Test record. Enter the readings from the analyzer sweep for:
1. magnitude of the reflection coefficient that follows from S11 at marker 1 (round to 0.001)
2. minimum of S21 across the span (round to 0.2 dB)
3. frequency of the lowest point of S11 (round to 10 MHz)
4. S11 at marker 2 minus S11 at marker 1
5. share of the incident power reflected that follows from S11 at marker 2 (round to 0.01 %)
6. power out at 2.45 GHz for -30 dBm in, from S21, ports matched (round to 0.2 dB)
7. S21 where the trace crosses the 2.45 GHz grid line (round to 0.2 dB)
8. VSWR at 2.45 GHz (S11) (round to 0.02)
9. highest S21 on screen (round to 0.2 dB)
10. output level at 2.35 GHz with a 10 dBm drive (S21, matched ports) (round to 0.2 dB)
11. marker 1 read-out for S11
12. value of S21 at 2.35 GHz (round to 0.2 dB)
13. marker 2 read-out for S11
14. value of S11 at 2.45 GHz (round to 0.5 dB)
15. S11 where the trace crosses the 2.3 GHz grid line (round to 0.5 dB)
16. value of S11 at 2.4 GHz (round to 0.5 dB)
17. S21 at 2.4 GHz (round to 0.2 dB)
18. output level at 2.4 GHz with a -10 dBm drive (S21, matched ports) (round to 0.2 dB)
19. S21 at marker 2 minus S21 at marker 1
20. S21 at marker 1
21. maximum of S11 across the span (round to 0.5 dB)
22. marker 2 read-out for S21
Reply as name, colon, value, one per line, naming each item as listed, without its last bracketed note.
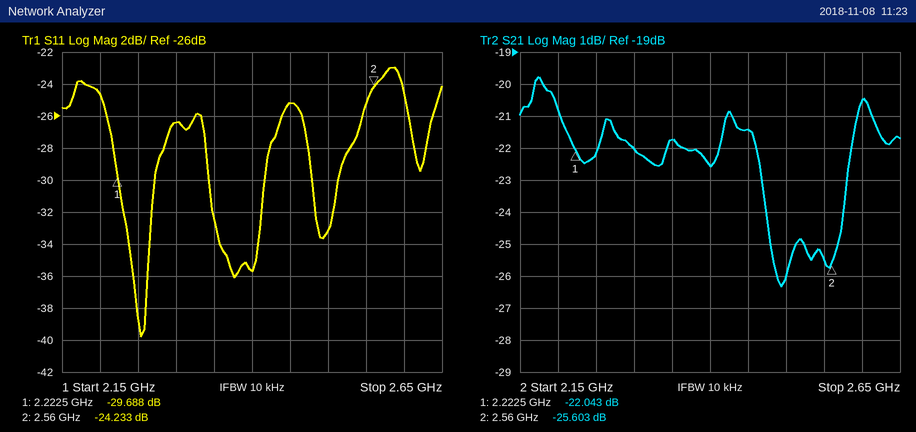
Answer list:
magnitude of the reflection coefficient that follows from S11 at marker 1: 0.033
minimum of S21 across the span: -26.4 dB
frequency of the lowest point of S11: 2.25 GHz
S11 at marker 2 minus S11 at marker 1: 5.455 dB
share of the incident power reflected that follows from S11 at marker 2: 0.38 %
power out at 2.45 GHz for -30 dBm in, from S21, ports matched: -51.4 dBm
S21 where the trace crosses the 2.45 GHz grid line: -21.4 dB
VSWR at 2.45 GHz (S11): 1.12
highest S21 on screen: -19.8 dB
output level at 2.35 GHz with a 10 dBm drive (S21, matched ports): -11.8 dBm
marker 1 read-out for S11: -29.688 dB
value of S21 at 2.35 GHz: -21.8 dB
marker 2 read-out for S11: -24.233 dB
value of S11 at 2.45 GHz: -25.0 dB
S11 where the trace crosses the 2.3 GHz grid line: -26.5 dB
value of S11 at 2.4 GHz: -35.5 dB
S21 at 2.4 GHz: -22.6 dB
output level at 2.4 GHz with a -10 dBm drive (S21, matched ports): -32.6 dBm
S21 at marker 2 minus S21 at marker 1: -3.560 dB
S21 at marker 1: -22.043 dB
maximum of S11 across the span: -23.0 dB
marker 2 read-out for S21: -25.603 dB
